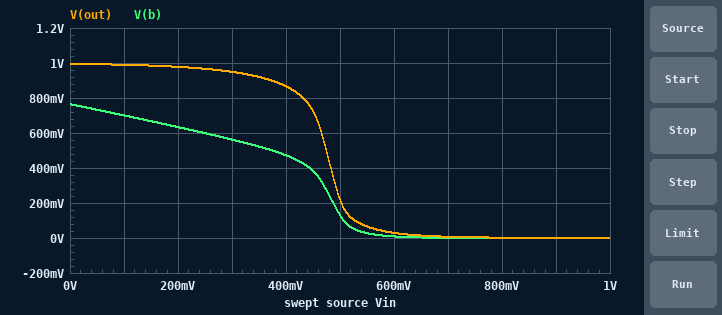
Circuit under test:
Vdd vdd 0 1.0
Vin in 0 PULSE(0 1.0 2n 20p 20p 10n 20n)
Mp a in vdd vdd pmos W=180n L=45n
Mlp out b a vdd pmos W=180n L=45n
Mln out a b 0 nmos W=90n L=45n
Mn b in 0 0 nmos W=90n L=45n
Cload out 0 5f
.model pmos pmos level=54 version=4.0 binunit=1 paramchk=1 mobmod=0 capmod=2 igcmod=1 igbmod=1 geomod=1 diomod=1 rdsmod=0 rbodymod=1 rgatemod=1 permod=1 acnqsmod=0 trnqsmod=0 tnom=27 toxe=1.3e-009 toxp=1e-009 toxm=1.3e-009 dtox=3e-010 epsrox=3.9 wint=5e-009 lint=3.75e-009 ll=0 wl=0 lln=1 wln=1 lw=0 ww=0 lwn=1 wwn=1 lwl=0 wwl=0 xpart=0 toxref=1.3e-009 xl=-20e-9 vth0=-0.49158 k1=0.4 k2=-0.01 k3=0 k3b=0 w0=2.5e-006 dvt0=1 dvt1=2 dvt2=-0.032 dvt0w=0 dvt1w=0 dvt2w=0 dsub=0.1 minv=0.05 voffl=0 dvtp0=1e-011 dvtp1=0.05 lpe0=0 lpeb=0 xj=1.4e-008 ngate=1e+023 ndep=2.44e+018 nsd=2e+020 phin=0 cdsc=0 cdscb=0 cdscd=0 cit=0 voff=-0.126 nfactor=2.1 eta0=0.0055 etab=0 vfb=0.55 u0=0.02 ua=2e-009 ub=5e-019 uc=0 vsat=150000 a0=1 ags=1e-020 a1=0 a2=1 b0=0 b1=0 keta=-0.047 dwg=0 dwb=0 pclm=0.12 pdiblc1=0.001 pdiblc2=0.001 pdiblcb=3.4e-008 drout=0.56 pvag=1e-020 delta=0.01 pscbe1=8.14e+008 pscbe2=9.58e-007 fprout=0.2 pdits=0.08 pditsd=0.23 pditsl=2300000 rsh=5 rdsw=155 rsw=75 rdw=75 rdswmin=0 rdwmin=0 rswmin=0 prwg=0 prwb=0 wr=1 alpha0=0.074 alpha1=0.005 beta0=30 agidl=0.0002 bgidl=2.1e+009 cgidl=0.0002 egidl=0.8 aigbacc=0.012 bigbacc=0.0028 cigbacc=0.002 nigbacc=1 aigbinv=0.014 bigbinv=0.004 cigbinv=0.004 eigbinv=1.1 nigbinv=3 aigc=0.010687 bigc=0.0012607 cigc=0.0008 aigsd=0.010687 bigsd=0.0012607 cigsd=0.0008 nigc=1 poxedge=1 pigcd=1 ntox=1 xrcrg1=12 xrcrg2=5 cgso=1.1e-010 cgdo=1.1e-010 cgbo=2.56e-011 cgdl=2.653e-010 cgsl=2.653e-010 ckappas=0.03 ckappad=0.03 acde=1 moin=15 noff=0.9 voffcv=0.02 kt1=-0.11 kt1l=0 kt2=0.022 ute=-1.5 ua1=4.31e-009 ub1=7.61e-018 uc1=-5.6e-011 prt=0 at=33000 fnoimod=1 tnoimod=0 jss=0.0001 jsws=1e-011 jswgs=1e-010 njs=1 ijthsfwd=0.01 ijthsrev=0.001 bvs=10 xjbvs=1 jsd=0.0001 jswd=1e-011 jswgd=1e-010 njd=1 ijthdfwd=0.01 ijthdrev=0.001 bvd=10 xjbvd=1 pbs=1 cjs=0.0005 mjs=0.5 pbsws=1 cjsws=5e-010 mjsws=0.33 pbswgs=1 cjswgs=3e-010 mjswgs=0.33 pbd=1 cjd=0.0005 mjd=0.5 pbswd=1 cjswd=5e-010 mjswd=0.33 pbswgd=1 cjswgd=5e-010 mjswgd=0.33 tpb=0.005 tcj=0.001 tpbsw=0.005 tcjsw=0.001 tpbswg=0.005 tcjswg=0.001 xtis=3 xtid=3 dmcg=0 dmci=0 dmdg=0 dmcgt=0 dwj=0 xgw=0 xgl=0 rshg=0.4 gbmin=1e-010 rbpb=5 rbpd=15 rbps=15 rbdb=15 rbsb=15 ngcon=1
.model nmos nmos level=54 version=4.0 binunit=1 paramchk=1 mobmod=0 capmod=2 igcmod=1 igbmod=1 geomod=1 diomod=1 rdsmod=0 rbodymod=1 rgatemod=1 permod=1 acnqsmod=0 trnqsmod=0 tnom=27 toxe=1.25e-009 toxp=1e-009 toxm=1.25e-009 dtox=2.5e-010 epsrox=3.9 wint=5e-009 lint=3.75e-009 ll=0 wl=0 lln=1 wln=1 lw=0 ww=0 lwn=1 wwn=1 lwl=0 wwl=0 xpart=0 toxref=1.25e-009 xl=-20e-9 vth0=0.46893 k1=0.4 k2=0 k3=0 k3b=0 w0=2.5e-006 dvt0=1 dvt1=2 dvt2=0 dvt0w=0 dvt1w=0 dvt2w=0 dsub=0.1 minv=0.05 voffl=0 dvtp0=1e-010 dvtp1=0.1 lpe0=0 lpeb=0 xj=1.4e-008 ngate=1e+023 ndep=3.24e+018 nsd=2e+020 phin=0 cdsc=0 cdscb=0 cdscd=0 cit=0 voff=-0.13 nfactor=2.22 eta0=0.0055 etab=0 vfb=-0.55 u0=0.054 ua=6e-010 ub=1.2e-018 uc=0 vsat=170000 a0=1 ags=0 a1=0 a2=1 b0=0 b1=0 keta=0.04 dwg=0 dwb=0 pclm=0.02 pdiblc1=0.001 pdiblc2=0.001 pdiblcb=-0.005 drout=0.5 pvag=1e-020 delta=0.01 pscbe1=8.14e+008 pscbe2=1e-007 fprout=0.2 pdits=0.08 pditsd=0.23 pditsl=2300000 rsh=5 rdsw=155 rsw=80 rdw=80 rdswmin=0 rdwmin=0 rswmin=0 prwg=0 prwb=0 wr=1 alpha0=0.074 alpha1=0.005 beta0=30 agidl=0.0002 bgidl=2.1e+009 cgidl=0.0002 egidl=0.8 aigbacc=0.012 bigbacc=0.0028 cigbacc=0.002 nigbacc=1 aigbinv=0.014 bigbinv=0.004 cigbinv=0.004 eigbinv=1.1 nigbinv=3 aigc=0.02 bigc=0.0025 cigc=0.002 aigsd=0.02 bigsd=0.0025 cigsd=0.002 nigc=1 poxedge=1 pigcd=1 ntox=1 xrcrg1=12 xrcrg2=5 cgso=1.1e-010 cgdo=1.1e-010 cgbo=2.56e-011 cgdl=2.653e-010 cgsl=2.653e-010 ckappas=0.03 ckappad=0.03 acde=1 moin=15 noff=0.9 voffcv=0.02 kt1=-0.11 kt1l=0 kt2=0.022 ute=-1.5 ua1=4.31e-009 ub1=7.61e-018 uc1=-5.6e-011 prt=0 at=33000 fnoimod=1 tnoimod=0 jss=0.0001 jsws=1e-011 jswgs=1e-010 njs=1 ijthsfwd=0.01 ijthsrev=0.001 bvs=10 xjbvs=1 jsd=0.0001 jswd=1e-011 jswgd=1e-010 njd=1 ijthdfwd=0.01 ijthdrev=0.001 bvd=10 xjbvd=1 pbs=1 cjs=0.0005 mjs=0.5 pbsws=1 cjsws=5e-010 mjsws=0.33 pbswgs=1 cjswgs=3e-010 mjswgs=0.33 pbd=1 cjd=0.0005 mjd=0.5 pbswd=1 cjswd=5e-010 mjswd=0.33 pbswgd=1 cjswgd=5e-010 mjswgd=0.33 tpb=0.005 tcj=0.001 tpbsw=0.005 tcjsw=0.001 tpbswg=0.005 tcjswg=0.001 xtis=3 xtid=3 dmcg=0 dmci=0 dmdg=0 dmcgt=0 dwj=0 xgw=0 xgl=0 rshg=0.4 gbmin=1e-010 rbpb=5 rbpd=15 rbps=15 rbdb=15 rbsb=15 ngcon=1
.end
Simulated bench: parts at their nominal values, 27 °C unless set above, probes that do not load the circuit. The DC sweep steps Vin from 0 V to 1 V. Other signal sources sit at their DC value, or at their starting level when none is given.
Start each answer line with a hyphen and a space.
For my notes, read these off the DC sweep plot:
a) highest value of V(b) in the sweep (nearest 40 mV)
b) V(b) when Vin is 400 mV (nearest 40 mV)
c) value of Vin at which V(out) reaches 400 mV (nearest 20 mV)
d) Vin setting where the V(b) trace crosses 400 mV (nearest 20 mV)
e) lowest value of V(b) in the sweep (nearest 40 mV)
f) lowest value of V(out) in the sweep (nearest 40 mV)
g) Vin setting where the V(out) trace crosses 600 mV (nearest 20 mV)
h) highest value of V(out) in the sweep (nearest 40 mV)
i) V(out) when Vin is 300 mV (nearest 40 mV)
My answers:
- 760 mV
- 480 mV
- 480 mV
- 440 mV
- 0 V
- 0 V
- 460 mV
- 1.00 V
- 960 mV
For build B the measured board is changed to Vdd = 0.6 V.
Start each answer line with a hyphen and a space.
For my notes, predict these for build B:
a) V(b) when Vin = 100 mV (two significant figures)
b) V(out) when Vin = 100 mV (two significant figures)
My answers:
- 380 mV
- 560 mV
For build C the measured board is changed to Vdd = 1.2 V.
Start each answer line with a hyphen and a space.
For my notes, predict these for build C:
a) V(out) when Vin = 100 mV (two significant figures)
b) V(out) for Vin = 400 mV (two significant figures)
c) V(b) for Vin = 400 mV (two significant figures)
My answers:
- 1.2 V
- 1.1 V
- 640 mV
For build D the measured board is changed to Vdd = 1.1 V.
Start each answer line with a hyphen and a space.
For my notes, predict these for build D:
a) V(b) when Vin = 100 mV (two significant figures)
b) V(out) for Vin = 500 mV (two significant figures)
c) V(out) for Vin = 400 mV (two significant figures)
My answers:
- 780 mV
- 800 mV
- 1.0 V
